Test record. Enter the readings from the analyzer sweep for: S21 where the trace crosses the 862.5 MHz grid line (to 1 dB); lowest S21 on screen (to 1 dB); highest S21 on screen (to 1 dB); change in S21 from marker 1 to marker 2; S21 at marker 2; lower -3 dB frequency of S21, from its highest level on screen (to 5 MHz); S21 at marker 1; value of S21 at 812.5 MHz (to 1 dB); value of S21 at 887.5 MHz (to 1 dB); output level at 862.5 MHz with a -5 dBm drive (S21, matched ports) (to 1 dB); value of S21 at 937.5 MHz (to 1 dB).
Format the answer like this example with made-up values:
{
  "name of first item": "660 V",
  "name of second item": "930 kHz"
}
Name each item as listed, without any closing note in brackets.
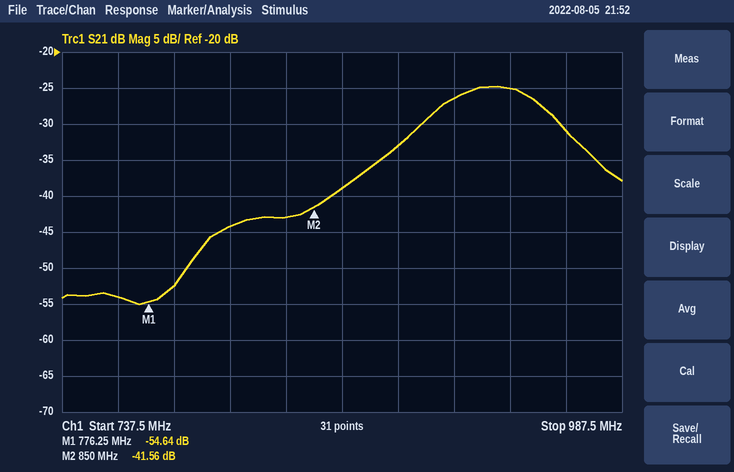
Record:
{
  "S21 where the trace crosses the 862.5 MHz grid line": "-39 dB",
  "lowest S21 on screen": "-55 dB",
  "highest S21 on screen": "-25 dB",
  "change in S21 from marker 1 to marker 2": "13.08 dB",
  "S21 at marker 2": "-41.56 dB",
  "lower -3 dB frequency of S21, from its highest level on screen": "905 MHz",
  "S21 at marker 1": "-54.64 dB",
  "value of S21 at 812.5 MHz": "-44 dB",
  "value of S21 at 887.5 MHz": "-33 dB",
  "output level at 862.5 MHz with a -5 dBm drive (S21, matched ports)": "-44 dBm",
  "value of S21 at 937.5 MHz": "-25 dB"
}
